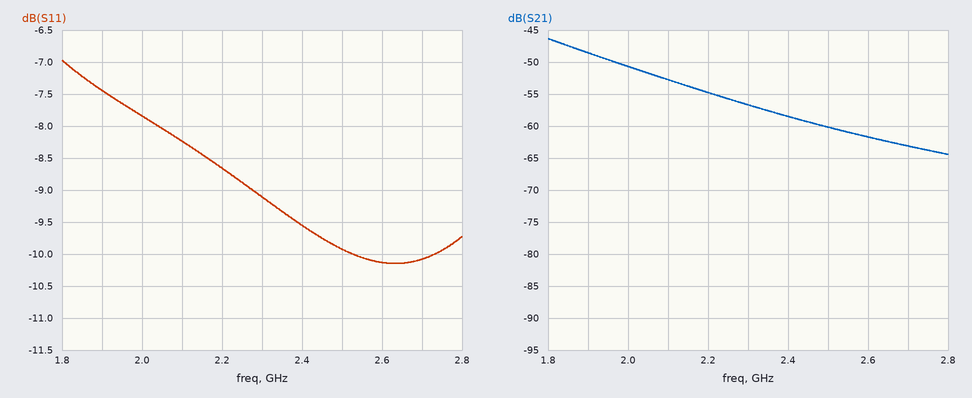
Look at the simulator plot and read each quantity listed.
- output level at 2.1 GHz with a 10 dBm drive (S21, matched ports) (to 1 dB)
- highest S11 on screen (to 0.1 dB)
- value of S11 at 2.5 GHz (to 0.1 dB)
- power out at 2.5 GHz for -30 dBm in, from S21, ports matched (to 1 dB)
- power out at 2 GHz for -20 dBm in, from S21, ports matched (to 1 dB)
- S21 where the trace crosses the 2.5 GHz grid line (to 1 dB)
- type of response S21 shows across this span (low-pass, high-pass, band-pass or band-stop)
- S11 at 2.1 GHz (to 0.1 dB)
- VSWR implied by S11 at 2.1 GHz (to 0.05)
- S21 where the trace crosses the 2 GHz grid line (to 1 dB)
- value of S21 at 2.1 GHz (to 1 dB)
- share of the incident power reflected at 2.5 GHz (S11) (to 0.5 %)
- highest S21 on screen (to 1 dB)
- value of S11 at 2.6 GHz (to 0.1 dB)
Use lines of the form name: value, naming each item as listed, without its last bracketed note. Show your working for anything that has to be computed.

output level at 2.1 GHz with a 10 dBm drive (S21, matched ports): 10 dBm + (-53 dB) = -43 dBm
highest S11 on screen: -7.0 dB
value of S11 at 2.5 GHz: -9.9 dB
power out at 2.5 GHz for -30 dBm in, from S21, ports matched: -30 dBm + (-60 dB) = -90 dBm
power out at 2 GHz for -20 dBm in, from S21, ports matched: -20 dBm + (-51 dB) = -71 dBm
S21 where the trace crosses the 2.5 GHz grid line: -60 dB
type of response S21 shows across this span: low-pass
S11 at 2.1 GHz: -8.2 dB
VSWR implied by S11 at 2.1 GHz: |Γ| = 10^(-8.2/20) = 0.3890; VSWR = (1 + 0.3890)/(1 − 0.3890) ≈ 2.27, so 2.25 to the nearest 0.05
S21 where the trace crosses the 2 GHz grid line: -51 dB
value of S21 at 2.1 GHz: -53 dB
share of the incident power reflected at 2.5 GHz (S11): 10^(-9.9/10) ≈ 10.2 %, so 10.0 % to the nearest 0.5 %
highest S21 on screen: -46 dB
value of S11 at 2.6 GHz: -10.1 dB
